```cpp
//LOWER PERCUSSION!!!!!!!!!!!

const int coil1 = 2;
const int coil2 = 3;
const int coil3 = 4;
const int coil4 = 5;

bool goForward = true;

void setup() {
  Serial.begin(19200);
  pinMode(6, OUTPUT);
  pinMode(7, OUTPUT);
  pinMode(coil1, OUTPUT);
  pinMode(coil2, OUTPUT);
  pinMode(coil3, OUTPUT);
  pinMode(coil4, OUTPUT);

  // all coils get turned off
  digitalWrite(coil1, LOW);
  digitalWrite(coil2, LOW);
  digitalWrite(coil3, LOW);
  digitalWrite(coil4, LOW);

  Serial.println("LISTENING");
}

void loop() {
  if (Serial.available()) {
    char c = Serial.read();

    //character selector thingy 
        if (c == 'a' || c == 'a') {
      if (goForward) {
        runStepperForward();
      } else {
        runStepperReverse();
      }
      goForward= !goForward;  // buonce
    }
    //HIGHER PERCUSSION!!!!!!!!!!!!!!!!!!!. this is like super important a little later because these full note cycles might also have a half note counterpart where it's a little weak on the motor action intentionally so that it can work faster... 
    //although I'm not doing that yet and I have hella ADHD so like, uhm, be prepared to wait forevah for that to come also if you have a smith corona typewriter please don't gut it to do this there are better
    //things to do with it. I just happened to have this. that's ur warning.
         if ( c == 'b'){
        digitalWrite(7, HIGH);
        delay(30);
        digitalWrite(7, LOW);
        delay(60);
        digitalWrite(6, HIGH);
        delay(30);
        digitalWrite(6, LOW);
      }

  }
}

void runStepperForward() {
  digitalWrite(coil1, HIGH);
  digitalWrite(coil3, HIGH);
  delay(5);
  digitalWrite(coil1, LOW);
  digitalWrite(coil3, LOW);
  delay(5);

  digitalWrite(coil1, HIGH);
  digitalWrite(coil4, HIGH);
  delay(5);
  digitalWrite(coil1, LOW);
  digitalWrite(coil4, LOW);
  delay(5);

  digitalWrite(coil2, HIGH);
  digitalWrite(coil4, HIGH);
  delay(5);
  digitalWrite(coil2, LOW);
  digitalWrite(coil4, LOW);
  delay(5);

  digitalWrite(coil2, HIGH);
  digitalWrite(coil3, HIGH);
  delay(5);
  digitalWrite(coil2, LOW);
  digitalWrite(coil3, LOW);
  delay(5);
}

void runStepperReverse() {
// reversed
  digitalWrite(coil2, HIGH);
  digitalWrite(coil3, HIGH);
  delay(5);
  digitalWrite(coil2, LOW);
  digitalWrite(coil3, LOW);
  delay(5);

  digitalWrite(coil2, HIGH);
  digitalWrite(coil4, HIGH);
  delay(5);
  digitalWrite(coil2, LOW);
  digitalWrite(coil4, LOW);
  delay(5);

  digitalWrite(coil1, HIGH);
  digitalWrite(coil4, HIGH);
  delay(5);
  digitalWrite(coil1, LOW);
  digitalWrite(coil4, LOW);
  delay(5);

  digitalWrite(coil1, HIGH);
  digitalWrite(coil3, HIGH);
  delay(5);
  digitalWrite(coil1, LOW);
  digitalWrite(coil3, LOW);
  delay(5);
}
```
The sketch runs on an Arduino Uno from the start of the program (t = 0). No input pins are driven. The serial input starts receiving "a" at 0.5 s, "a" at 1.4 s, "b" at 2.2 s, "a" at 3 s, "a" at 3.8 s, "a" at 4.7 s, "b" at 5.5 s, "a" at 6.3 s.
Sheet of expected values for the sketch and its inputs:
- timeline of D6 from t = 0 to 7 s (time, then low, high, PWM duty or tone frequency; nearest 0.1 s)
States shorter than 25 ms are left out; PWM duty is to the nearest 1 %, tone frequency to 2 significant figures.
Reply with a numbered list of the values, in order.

1. 0 s low; 2.3 s high; 2.3 s low; 5.6 s high; 5.6 s low
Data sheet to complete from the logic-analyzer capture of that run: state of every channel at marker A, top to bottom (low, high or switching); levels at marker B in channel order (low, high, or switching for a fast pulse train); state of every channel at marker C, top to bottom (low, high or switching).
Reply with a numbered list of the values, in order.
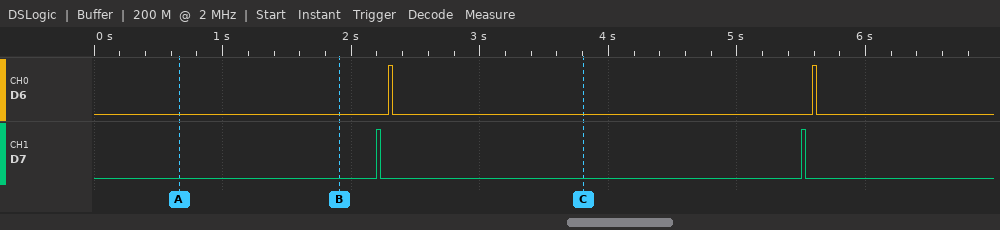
1. D6 low, D7 low
2. D6 low, D7 low
3. D6 low, D7 low
